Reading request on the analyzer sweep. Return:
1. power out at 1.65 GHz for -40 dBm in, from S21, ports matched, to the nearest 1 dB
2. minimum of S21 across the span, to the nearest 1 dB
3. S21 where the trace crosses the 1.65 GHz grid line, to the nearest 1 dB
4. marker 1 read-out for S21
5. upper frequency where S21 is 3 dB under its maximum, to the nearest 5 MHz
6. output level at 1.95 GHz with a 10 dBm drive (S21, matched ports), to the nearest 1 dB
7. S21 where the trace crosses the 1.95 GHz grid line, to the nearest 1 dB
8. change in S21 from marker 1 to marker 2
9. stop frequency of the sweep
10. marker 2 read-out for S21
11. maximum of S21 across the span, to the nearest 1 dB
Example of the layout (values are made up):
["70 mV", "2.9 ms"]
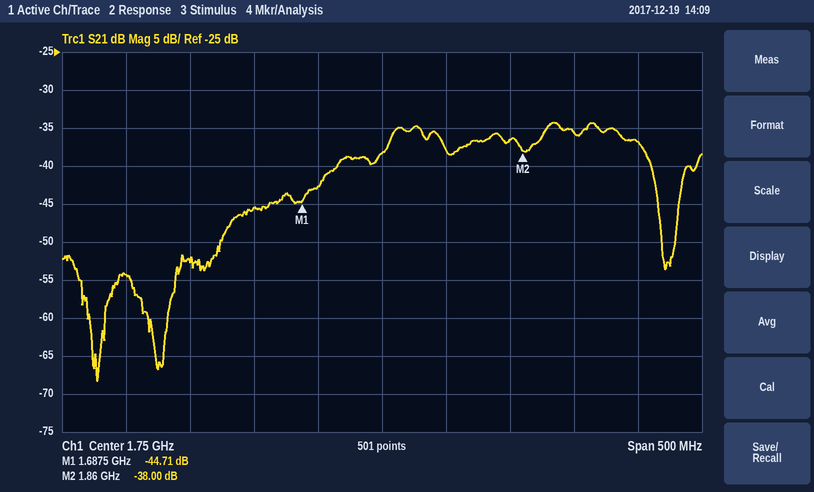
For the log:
["-85 dBm", "-68 dB", "-45 dB", "-44.71 dB", "1.950 GHz", "-27 dBm", "-37 dB", "6.71 dB", "2 GHz", "-38.00 dB", "-34 dB"]
